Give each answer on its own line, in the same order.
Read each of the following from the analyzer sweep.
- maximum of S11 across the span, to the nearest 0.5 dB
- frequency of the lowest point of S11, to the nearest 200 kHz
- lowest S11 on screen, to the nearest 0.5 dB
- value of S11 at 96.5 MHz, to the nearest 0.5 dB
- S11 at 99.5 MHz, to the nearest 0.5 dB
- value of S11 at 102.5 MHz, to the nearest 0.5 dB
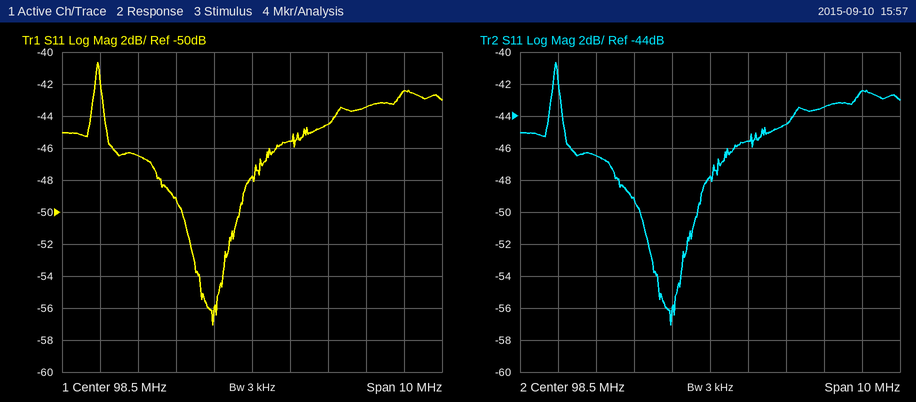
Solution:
-40.5 dB
97.4 MHz
-57.0 dB
-49.0 dB
-45.5 dB
-42.5 dB
